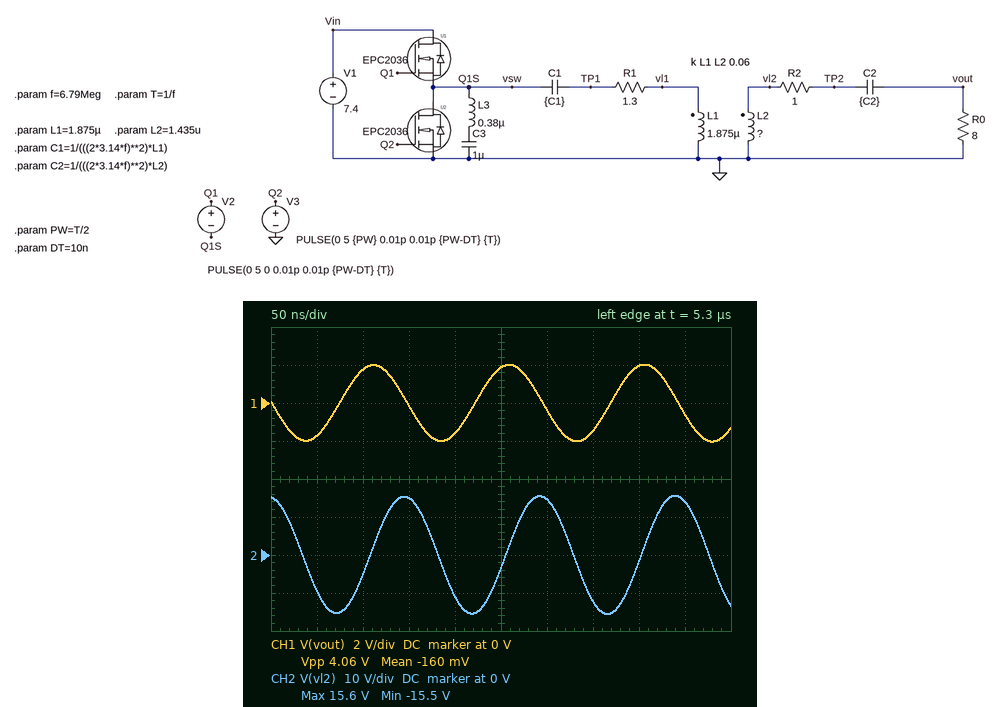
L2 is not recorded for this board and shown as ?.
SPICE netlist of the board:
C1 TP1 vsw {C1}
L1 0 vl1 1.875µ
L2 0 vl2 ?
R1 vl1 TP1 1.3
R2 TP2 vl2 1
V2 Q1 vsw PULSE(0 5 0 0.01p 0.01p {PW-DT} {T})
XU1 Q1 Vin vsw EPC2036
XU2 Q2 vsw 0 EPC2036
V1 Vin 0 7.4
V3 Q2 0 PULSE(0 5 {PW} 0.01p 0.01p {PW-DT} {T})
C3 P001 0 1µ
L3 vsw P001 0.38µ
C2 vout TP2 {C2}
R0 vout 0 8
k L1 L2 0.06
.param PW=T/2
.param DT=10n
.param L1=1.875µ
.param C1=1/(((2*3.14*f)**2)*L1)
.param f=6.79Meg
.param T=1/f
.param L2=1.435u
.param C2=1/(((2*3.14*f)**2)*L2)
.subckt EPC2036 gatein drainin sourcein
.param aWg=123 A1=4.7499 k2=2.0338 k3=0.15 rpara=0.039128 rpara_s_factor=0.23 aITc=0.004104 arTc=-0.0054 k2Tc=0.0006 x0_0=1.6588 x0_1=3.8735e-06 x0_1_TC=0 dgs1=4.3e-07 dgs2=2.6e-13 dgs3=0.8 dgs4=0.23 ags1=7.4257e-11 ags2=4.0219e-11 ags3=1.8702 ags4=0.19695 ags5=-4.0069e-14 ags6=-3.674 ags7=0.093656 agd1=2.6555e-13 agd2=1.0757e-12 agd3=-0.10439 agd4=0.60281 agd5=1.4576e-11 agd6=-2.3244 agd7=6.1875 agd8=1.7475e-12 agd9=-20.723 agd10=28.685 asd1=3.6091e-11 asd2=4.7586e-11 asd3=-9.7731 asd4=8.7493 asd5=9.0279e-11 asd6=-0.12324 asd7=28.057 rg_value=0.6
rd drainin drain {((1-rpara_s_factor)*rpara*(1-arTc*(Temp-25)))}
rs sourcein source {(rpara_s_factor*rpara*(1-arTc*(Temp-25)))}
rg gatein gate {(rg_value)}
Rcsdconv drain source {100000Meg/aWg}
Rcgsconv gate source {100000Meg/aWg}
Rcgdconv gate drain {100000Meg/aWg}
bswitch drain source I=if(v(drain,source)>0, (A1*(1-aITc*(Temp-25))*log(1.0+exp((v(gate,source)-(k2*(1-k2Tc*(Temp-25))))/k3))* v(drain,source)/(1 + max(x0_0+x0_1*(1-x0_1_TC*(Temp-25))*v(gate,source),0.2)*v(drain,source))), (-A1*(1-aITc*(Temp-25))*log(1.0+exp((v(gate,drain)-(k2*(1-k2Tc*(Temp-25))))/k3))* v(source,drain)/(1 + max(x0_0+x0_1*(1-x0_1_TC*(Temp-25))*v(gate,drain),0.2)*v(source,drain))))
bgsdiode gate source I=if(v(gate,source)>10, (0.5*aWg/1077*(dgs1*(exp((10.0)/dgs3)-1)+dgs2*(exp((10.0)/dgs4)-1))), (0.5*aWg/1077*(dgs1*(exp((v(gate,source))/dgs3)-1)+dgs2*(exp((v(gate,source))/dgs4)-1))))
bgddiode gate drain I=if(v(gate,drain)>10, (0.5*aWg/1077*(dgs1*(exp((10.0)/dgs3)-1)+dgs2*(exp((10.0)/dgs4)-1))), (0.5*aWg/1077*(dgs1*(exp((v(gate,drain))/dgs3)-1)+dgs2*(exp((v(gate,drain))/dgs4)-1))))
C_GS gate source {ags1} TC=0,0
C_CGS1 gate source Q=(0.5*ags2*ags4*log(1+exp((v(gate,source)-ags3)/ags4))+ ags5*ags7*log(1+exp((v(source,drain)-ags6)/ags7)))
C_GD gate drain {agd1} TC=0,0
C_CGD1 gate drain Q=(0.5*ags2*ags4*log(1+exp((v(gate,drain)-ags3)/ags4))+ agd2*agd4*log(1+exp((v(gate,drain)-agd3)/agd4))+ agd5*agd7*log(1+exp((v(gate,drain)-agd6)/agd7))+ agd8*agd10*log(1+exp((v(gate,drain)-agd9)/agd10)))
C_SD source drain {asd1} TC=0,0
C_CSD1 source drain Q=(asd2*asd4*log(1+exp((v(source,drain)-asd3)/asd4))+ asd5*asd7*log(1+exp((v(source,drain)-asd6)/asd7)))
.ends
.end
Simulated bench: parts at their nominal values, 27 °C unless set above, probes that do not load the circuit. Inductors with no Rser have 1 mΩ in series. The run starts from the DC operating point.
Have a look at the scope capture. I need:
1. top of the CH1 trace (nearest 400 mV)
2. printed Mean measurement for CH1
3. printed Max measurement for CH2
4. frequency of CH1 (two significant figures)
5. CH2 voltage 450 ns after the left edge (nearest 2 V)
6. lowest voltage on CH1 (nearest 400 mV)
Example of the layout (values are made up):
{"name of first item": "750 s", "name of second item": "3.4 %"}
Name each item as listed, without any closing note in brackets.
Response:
{"top of the CH1 trace": "2.0 V", "printed Mean measurement for CH1": "-160 mV", "printed Max measurement for CH2": "15.6 V", "frequency of CH1": "6.8 MHz", "CH2 voltage 450 ns after the left edge": "14 V", "lowest voltage on CH1": "-2.0 V"}
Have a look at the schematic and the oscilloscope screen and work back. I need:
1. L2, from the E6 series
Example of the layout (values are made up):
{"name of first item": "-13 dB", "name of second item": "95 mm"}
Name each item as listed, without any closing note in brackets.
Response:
{"L2, from the E6 series": "680 nH"}
